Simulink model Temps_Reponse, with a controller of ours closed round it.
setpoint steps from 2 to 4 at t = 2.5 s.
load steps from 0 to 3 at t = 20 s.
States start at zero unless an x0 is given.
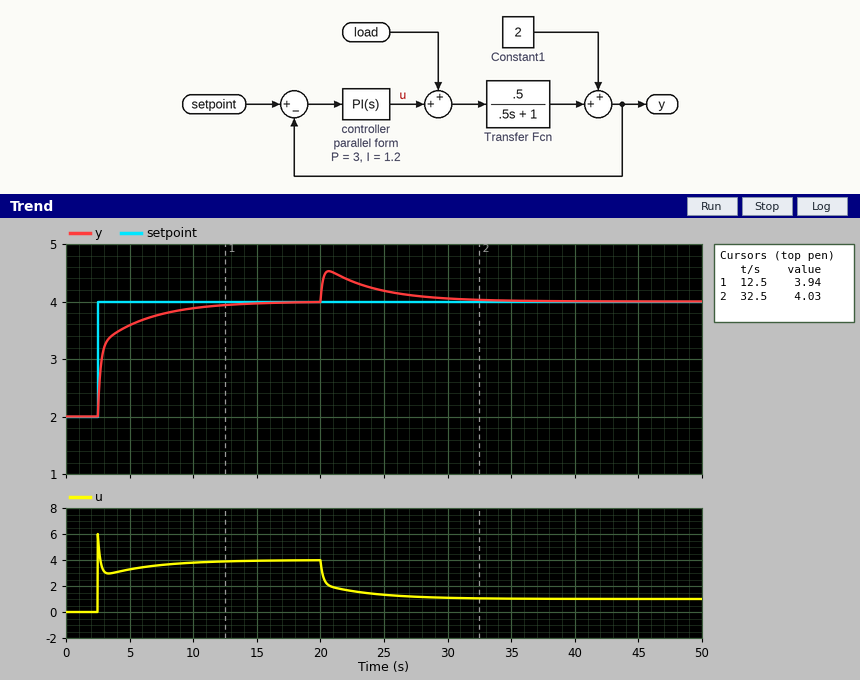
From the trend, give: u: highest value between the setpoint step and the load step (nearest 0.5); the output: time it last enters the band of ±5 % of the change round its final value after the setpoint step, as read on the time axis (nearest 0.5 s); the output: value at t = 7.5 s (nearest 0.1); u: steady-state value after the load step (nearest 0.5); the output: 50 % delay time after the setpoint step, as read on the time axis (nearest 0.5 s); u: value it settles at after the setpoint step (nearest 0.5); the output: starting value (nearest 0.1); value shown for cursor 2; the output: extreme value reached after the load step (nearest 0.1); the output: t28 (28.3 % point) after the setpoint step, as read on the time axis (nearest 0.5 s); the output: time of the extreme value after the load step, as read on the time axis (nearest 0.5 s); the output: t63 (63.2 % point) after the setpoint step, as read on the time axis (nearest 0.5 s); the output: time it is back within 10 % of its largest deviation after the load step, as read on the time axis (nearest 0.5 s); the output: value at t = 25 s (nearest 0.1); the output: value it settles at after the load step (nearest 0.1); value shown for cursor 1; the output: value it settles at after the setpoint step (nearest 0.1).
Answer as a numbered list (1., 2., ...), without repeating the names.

1. 6.0
2. 10.5 s
3. 3.8
4. 1.0
5. 3.0 s
6. 4.0
7. 2.0
8. 4.03
9. 4.5
10. 2.5 s
11. 20.5 s
12. 3.0 s
13. 30.0 s
14. 4.2
15. 4.0
16. 3.94
17. 4.0
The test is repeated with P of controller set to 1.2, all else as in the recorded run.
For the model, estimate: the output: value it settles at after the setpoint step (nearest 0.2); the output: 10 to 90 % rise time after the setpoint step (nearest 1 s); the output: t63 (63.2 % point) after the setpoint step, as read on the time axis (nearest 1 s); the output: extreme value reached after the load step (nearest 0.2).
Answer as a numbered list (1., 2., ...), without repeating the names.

1. 4.0
2. 4 s
3. 4 s
4. 4.8
